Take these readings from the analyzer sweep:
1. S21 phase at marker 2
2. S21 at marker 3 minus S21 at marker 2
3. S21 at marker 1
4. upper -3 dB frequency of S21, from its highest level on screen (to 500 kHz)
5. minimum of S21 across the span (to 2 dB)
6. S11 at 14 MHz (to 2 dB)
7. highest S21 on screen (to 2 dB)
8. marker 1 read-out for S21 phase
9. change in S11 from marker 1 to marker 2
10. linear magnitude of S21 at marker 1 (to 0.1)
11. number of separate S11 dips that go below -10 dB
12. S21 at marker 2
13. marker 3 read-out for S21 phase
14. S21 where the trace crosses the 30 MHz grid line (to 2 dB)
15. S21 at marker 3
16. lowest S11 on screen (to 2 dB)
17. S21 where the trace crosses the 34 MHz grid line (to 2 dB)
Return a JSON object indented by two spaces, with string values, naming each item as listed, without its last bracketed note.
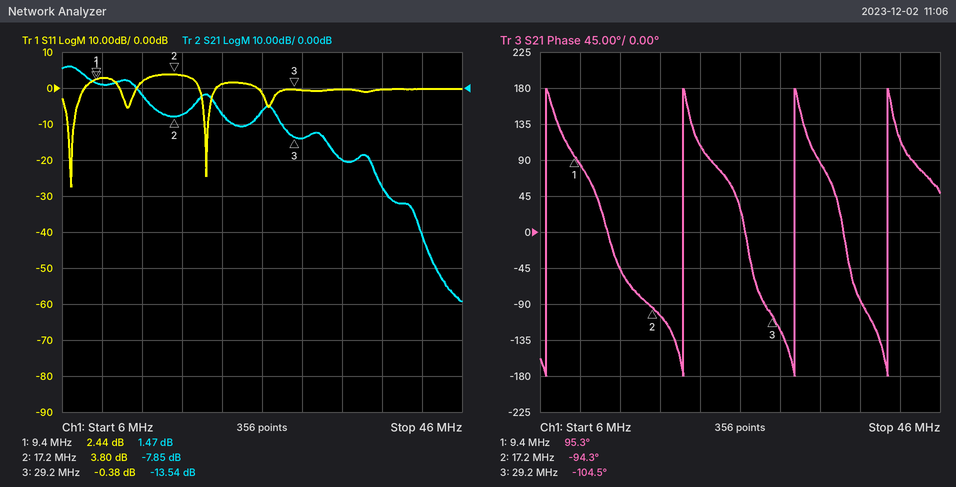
{
  "S21 phase at marker 2": "-94.3°",
  "S21 at marker 3 minus S21 at marker 2": "-5.69 dB",
  "S21 at marker 1": "1.47 dB",
  "upper -3 dB frequency of S21, from its highest level on screen": "8.5 MHz",
  "minimum of S21 across the span": "-60 dB",
  "S11 at 14 MHz": "2 dB",
  "highest S21 on screen": "6 dB",
  "marker 1 read-out for S21 phase": "95.3°",
  "change in S11 from marker 1 to marker 2": "1.36 dB",
  "linear magnitude of S21 at marker 1": "1.2",
  "number of separate S11 dips that go below -10 dB": "2",
  "S21 at marker 2": "-7.85 dB",
  "marker 3 read-out for S21 phase": "-104.5°",
  "S21 where the trace crosses the 30 MHz grid line": "-14 dB",
  "S21 at marker 3": "-13.54 dB",
  "lowest S11 on screen": "-28 dB",
  "S21 where the trace crosses the 34 MHz grid line": "-20 dB"
}
